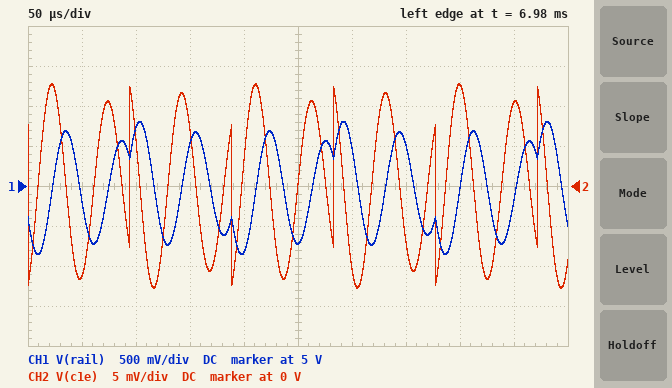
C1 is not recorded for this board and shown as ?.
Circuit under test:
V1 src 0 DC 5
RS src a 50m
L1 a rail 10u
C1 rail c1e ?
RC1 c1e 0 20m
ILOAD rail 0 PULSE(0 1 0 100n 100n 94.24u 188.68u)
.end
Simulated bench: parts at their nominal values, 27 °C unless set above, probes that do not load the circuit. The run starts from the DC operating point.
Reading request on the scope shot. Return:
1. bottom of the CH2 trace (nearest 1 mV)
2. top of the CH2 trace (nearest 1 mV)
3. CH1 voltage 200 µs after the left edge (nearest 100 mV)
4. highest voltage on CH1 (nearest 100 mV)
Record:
-13 mV
13 mV
4.2 V
5.8 V
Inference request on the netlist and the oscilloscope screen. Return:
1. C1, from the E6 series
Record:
6.8 µF
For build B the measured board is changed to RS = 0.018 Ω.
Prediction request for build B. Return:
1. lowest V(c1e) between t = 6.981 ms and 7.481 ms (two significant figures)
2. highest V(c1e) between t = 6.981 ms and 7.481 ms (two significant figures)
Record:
-12 mV
12 mV
